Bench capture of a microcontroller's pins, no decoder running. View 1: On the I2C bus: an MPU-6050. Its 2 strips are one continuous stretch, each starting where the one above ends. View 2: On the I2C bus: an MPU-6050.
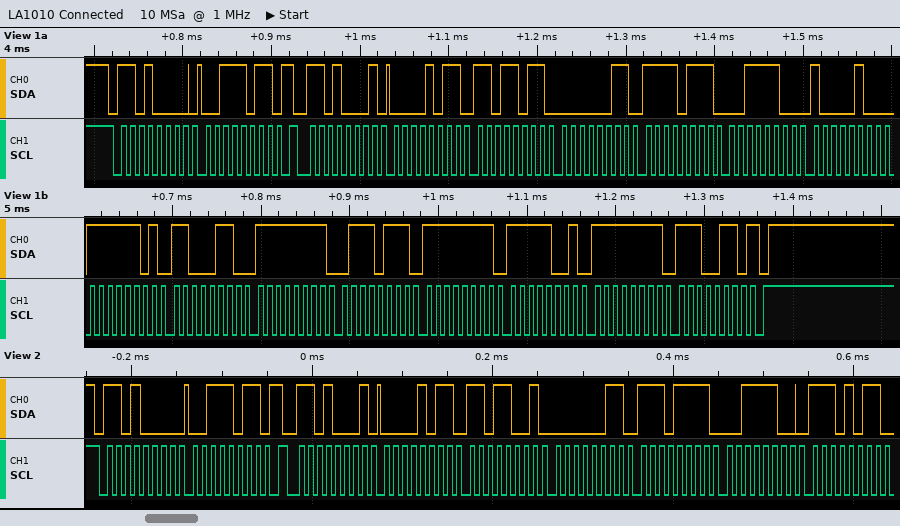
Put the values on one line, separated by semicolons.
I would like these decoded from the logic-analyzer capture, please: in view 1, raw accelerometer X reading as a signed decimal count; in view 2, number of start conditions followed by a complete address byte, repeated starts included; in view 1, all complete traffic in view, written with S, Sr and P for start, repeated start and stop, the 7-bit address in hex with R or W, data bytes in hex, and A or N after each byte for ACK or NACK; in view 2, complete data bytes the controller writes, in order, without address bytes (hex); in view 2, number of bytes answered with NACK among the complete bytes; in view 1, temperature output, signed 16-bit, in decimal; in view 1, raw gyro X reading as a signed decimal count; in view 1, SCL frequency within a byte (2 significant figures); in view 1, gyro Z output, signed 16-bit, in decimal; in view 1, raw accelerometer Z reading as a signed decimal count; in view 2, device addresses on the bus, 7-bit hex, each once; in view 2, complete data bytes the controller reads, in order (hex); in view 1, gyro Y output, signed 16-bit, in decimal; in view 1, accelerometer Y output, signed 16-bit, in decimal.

3035; 2; S 68W A 3B A Sr 68R A 0B A DB A 03 A F7 A 3C A 84 A FD A C6 A FF A 77 A FF A F9 A FF A E6 N P; 3B; 0; -570; -137; 100 kHz; -26; 15492; 0x68; 0B D9 03 EF 3C EB; -7; 1015
